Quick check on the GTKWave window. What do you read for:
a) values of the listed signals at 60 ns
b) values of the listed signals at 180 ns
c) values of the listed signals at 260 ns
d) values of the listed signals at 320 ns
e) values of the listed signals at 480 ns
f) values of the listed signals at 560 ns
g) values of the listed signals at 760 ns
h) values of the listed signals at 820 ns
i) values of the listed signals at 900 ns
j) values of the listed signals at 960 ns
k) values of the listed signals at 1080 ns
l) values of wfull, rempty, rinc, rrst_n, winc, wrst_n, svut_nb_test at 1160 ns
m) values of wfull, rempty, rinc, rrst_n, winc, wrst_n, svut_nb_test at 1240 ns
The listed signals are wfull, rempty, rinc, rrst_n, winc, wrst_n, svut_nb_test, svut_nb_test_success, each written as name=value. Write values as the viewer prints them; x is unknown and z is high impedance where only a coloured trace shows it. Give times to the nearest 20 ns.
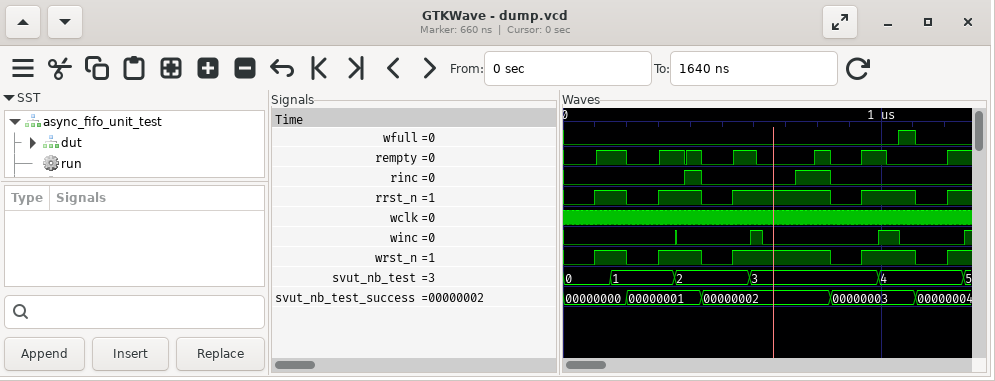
wfull=0, rempty=0, rinc=0, rrst_n=0, winc=0, wrst_n=0, svut_nb_test=0, svut_nb_test_success=00000000
wfull=0, rempty=1, rinc=0, rrst_n=1, winc=0, wrst_n=1, svut_nb_test=1, svut_nb_test_success=00000000
wfull=0, rempty=0, rinc=0, rrst_n=0, winc=0, wrst_n=0, svut_nb_test=1, svut_nb_test_success=00000001
wfull=0, rempty=1, rinc=0, rrst_n=1, winc=0, wrst_n=1, svut_nb_test=1, svut_nb_test_success=00000001
wfull=0, rempty=0, rinc=0, rrst_n=0, winc=0, wrst_n=0, svut_nb_test=2, svut_nb_test_success=00000002
wfull=0, rempty=1, rinc=0, rrst_n=1, winc=0, wrst_n=1, svut_nb_test=2, svut_nb_test_success=00000002
wfull=0, rempty=0, rinc=1, rrst_n=1, winc=0, wrst_n=1, svut_nb_test=3, svut_nb_test_success=00000002
wfull=0, rempty=1, rinc=1, rrst_n=1, winc=0, wrst_n=1, svut_nb_test=3, svut_nb_test_success=00000002
wfull=0, rempty=0, rinc=0, rrst_n=0, winc=0, wrst_n=0, svut_nb_test=3, svut_nb_test_success=00000003
wfull=0, rempty=1, rinc=0, rrst_n=1, winc=0, wrst_n=1, svut_nb_test=3, svut_nb_test_success=00000003
wfull=1, rempty=0, rinc=0, rrst_n=1, winc=0, wrst_n=1, svut_nb_test=4, svut_nb_test_success=00000003
wfull=0, rempty=0, rinc=0, rrst_n=0, winc=0, wrst_n=0, svut_nb_test=4
wfull=0, rempty=1, rinc=0, rrst_n=1, winc=0, wrst_n=1, svut_nb_test=4
